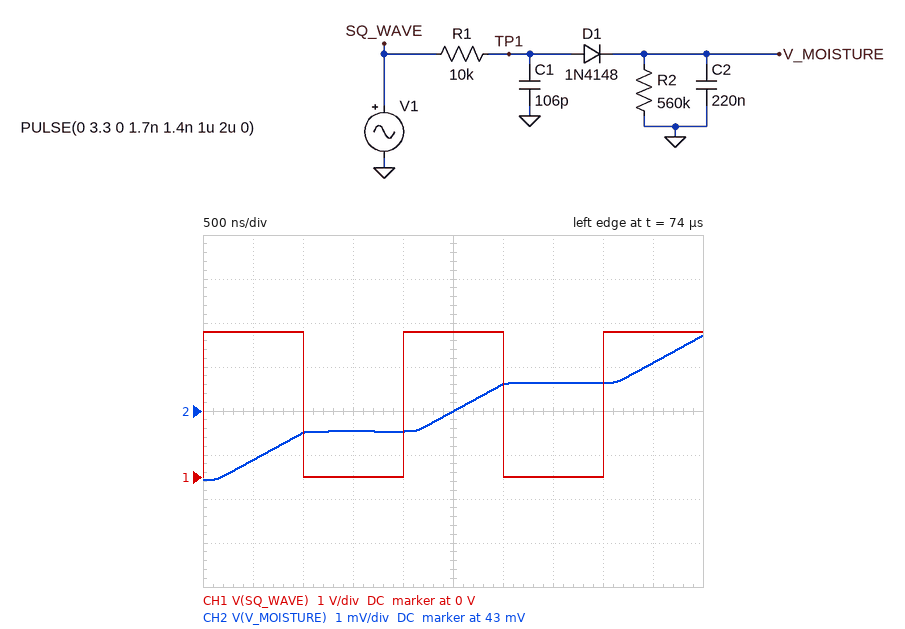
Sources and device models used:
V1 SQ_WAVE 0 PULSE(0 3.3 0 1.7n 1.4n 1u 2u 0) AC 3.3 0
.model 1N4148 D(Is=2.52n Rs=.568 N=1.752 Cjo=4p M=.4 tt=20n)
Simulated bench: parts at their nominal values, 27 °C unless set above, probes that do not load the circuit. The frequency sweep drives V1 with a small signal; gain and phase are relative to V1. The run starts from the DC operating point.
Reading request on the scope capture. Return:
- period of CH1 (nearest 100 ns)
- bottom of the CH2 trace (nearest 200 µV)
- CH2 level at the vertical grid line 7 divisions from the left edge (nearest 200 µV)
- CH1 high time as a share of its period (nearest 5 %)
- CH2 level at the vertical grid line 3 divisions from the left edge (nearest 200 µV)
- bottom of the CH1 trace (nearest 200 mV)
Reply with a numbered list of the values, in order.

1. 2.0 µs
2. 41.4 mV
3. 43.6 mV
4. 50 %
5. 42.6 mV
6. 0 V
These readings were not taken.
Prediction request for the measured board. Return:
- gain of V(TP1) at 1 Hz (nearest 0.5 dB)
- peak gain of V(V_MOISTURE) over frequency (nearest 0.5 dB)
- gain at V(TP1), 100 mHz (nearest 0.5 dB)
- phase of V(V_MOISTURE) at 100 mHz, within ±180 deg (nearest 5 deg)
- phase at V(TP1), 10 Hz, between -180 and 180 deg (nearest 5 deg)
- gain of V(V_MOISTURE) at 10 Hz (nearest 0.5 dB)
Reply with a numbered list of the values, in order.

1. 0 dB
2. -30.5 dB
3. 0 dB
4. -5 deg
5. 0 deg
6. -48.0 dB
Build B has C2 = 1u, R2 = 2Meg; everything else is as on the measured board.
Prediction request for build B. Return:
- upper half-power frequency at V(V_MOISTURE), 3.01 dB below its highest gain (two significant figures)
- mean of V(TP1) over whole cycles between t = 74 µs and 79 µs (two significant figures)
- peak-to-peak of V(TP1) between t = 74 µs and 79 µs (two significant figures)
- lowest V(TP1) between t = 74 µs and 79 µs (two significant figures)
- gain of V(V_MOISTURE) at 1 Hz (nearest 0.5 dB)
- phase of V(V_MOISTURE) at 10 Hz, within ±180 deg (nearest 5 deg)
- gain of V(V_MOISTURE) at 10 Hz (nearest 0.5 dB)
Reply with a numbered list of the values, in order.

1. 88 mHz
2. 410 mV
3. 350 mV
4. 180 mV
5. -41.0 dB
6. -90 deg
7. -61.0 dB
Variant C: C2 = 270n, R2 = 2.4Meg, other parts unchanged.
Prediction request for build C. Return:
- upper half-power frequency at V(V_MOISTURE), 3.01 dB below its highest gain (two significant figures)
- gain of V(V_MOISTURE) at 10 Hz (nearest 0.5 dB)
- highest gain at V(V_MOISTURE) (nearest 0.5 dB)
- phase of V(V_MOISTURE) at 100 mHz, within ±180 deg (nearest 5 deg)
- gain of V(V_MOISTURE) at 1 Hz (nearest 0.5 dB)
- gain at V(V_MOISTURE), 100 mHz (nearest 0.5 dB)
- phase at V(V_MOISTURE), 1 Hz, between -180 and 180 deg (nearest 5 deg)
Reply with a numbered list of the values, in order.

1. 280 mHz
2. -49.5 dB
3. -18.5 dB
4. -20 deg
5. -30.0 dB
6. -19.0 dB
7. -75 deg
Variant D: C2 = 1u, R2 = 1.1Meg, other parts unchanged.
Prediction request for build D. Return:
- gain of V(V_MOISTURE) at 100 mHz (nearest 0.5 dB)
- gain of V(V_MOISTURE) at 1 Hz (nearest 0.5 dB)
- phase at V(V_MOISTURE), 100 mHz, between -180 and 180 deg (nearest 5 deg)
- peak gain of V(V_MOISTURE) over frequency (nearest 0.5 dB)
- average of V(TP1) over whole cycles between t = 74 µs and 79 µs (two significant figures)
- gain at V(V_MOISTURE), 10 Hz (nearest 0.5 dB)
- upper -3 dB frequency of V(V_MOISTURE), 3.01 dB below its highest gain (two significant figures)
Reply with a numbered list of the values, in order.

1. -26.5 dB
2. -41.0 dB
3. -35 deg
4. -25.0 dB
5. 410 mV
6. -61.0 dB
7. 150 mHz
